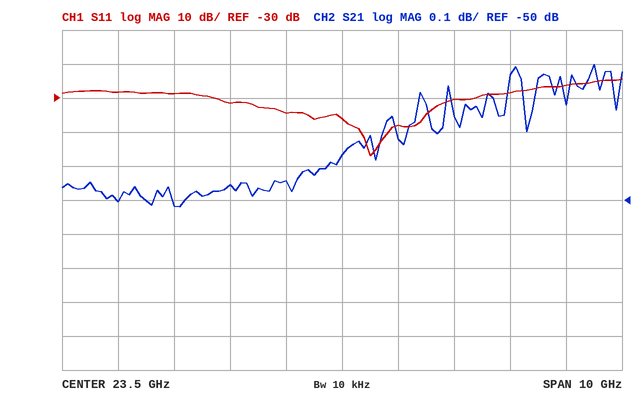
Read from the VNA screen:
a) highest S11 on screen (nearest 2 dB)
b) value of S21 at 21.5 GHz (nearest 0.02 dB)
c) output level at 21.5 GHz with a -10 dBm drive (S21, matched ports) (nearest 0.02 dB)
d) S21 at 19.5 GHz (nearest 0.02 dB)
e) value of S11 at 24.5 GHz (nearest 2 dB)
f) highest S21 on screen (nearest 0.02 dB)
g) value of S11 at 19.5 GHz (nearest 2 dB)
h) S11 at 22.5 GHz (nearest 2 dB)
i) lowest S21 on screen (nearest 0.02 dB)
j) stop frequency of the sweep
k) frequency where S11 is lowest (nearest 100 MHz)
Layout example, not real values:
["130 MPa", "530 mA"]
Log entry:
["-24 dB", "-49.96 dB", "-59.96 dBm", "-50.00 dB", "-38 dB", "-49.60 dB", "-28 dB", "-34 dB", "-50.02 dB", "28.5 GHz", "24.0 GHz"]
